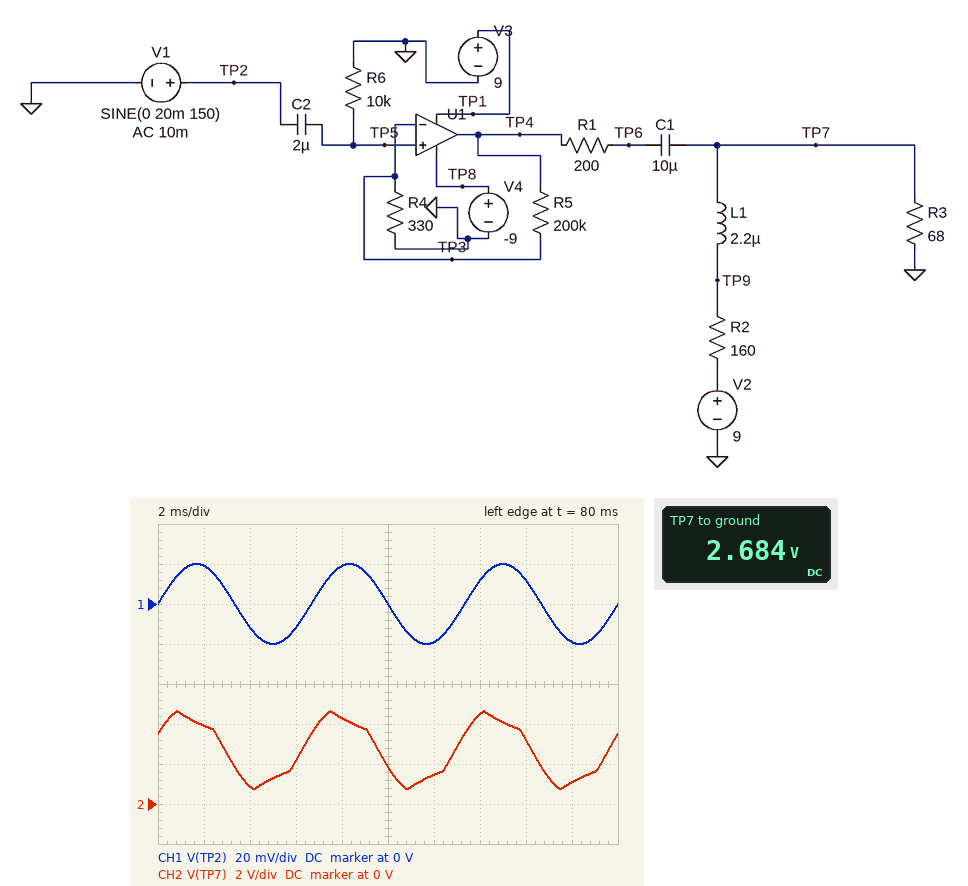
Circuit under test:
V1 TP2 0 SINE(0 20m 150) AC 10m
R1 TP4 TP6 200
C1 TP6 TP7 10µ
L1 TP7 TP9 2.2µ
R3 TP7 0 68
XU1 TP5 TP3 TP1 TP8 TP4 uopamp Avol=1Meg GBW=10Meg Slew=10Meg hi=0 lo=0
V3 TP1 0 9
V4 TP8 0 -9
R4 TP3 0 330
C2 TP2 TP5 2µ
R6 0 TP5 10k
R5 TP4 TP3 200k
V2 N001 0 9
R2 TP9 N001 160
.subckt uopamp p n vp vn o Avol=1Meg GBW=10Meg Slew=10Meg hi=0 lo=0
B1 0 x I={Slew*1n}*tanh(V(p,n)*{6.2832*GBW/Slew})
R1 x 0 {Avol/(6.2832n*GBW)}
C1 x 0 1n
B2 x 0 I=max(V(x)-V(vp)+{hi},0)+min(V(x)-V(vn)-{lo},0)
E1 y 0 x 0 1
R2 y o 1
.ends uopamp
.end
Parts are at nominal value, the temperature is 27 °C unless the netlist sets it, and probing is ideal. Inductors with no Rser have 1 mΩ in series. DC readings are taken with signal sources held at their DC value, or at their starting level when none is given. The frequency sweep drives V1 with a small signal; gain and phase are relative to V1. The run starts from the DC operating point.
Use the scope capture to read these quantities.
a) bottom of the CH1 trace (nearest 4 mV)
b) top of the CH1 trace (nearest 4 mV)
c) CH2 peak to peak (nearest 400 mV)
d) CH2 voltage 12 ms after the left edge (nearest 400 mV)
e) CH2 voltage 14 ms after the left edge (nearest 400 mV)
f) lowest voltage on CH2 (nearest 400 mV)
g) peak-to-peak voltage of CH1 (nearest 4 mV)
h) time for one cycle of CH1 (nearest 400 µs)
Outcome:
-20 mV
20 mV
4.0 V
1.6 V
4.4 V
800 mV
40 mV
6.8 ms
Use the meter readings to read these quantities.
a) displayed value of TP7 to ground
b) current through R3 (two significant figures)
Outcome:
2.684 V
39 mA
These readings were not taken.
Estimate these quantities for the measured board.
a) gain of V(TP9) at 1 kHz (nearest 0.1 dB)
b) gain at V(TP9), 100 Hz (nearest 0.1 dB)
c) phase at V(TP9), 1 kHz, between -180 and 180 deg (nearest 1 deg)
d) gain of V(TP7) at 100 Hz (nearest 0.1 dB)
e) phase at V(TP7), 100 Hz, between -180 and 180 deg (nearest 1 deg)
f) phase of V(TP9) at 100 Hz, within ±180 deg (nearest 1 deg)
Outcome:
41.3 dB
39.8 dB
1 deg
39.8 dB
37 deg
37 deg
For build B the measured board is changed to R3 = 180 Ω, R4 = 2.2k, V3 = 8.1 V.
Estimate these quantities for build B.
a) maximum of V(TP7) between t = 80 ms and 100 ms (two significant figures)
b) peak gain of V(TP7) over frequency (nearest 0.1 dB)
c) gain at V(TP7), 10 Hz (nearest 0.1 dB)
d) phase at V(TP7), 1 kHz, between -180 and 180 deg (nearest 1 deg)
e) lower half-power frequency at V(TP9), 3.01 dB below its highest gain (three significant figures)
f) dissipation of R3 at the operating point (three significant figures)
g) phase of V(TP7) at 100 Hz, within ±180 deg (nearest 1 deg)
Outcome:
5.3 V
28.7 dB
11.5 dB
3 deg
56.9 Hz
126 mW
34 deg
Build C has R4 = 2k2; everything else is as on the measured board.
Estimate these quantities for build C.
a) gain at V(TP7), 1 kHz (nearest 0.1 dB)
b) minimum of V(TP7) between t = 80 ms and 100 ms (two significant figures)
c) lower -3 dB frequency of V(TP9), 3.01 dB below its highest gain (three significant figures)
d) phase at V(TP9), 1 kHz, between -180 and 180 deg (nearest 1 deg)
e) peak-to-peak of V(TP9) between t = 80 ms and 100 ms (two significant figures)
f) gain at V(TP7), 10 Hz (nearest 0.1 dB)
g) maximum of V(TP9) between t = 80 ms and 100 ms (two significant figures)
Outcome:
24.9 dB
2.4 V
65.1 Hz
4 deg
650 mV
6.6 dB
3.0 V
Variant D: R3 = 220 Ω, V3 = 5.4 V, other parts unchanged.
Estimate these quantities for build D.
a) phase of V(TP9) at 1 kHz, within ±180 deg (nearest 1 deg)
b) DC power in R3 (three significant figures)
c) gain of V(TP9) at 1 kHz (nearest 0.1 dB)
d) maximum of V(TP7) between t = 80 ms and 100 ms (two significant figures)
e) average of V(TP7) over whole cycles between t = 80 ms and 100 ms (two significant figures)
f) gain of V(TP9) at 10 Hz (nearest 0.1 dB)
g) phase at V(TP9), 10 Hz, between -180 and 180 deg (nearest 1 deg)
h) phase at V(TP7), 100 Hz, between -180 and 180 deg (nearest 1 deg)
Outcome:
0 deg
123 mW
45.6 dB
7.8 V
5.2 V
28.7 dB
118 deg
33 deg
